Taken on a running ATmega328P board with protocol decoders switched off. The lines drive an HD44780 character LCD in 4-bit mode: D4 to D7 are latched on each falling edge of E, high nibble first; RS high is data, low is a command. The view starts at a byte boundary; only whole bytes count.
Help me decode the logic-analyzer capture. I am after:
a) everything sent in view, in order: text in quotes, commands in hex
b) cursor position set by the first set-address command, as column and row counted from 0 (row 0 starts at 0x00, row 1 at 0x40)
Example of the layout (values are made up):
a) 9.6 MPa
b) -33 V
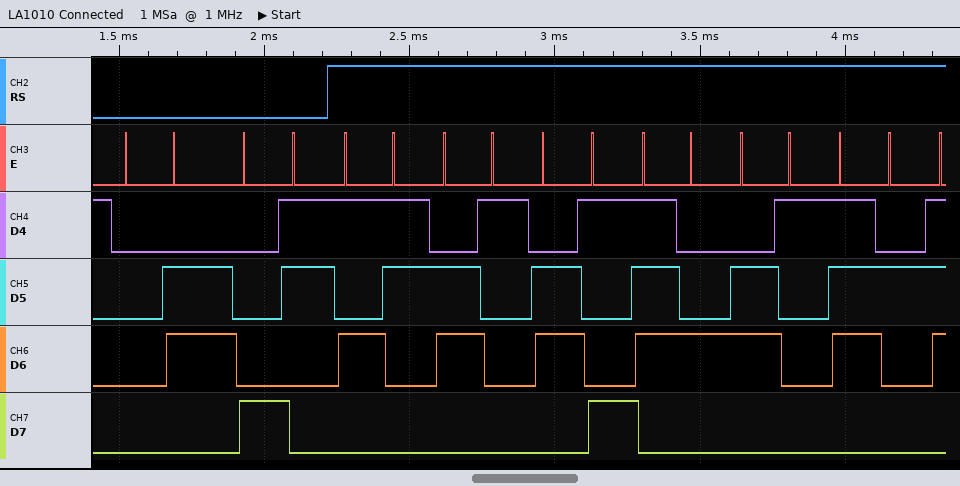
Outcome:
a) 0x06 0x83 "Saitar"
b) column 3, row 0
